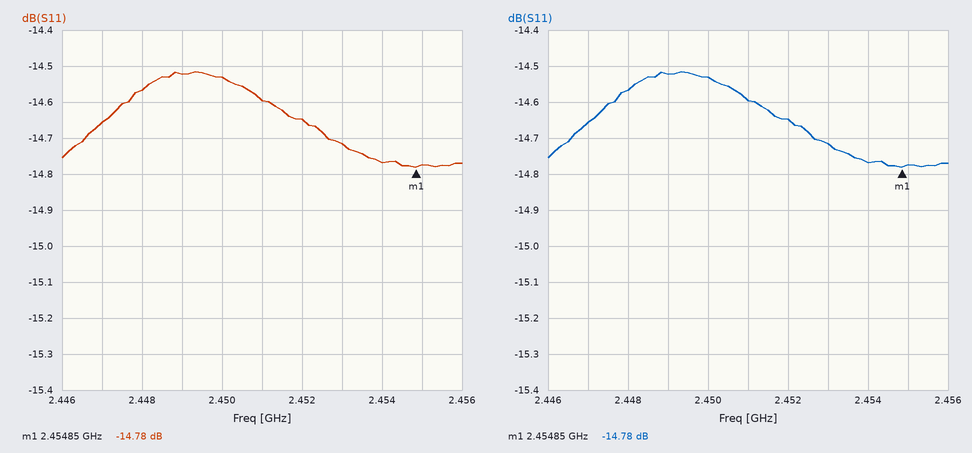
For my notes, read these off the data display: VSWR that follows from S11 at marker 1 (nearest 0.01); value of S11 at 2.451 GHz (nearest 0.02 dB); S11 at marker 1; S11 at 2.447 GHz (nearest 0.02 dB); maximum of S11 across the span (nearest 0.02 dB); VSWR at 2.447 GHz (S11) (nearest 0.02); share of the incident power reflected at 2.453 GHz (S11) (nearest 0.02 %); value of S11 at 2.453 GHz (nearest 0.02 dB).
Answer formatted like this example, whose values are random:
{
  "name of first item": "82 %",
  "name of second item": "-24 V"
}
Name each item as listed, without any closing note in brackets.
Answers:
{
  "VSWR that follows from S11 at marker 1": "1.45",
  "value of S11 at 2.451 GHz": "-14.60 dB",
  "S11 at marker 1": "-14.78 dB",
  "S11 at 2.447 GHz": "-14.66 dB",
  "maximum of S11 across the span": "-14.52 dB",
  "VSWR at 2.447 GHz (S11)": "1.46",
  "share of the incident power reflected at 2.453 GHz (S11)": "3.38 %",
  "value of S11 at 2.453 GHz": "-14.72 dB"
}
